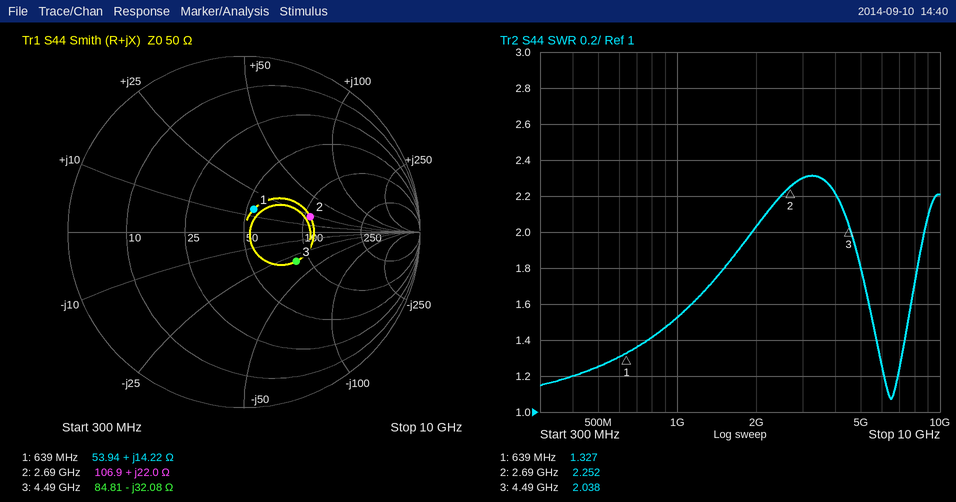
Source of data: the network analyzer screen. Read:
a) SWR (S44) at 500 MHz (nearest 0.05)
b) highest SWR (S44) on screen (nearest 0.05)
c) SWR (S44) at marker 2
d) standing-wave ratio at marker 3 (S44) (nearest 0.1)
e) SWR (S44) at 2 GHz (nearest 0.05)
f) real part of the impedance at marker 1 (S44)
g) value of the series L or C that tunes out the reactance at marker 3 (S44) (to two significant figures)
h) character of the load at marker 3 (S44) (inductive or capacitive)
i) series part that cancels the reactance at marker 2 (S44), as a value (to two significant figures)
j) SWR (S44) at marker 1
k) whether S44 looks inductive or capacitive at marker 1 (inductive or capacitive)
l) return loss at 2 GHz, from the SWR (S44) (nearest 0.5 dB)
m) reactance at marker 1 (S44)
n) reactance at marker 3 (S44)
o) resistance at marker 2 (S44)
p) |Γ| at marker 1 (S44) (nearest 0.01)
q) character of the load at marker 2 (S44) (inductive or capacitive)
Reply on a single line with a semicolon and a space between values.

1.25; 2.30; 2.252; 2.0; 2.05; 53.94 Ω; 1.1 nH; capacitive; 2.7 pF; 1.327; inductive; 9.5 dB; +14.22 Ω; -32.08 Ω; 106.9 Ω; 0.14; inductive
